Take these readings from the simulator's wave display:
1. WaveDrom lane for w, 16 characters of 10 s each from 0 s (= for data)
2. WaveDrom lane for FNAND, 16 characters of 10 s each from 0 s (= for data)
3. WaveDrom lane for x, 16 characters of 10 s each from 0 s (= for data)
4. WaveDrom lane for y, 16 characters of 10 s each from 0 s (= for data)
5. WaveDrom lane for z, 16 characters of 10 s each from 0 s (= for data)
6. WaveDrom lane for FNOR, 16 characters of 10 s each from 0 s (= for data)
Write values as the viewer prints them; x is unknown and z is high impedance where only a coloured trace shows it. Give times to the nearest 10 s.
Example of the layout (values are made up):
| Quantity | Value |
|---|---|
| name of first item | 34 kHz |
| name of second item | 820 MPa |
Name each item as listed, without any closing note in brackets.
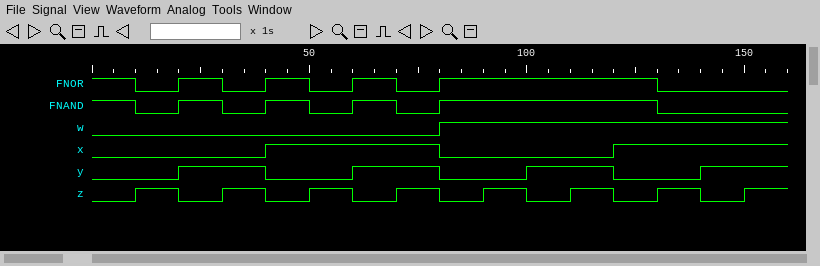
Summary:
| Quantity | Value |
|---|---|
| WaveDrom lane for w, 16 characters of 10 s each from 0 s | {name: 'w', wave: '0.......1.......'} |
| WaveDrom lane for FNAND, 16 characters of 10 s each from 0 s | {name: 'FNAND', wave: '101010101....0..'} |
| WaveDrom lane for x, 16 characters of 10 s each from 0 s | {name: 'x', wave: '0...1...0...1...'} |
| WaveDrom lane for y, 16 characters of 10 s each from 0 s | {name: 'y', wave: '0.1.0.1.0.1.0.1.'} |
| WaveDrom lane for z, 16 characters of 10 s each from 0 s | {name: 'z', wave: '0101010101010101'} |
| WaveDrom lane for FNOR, 16 characters of 10 s each from 0 s | {name: 'FNOR', wave: '101010101....0..'} |
